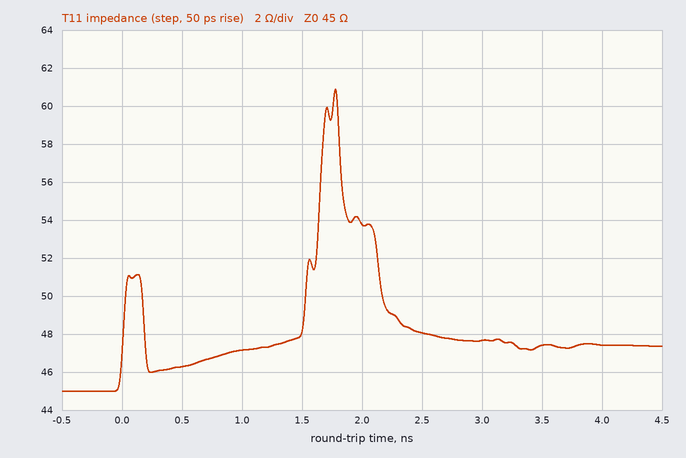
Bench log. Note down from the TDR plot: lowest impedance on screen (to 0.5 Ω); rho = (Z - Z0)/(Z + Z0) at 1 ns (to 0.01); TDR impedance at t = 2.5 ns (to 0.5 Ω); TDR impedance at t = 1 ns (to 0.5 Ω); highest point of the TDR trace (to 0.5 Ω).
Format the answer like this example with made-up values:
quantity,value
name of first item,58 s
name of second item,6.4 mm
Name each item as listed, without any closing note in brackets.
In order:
quantity,value
lowest impedance on screen,45.0 Ω
rho = (Z - Z0)/(Z + Z0) at 1 ns,+0.02
TDR impedance at t = 2.5 ns,48.0 Ω
TDR impedance at t = 1 ns,47.0 Ω
highest point of the TDR trace,61.0 Ω
